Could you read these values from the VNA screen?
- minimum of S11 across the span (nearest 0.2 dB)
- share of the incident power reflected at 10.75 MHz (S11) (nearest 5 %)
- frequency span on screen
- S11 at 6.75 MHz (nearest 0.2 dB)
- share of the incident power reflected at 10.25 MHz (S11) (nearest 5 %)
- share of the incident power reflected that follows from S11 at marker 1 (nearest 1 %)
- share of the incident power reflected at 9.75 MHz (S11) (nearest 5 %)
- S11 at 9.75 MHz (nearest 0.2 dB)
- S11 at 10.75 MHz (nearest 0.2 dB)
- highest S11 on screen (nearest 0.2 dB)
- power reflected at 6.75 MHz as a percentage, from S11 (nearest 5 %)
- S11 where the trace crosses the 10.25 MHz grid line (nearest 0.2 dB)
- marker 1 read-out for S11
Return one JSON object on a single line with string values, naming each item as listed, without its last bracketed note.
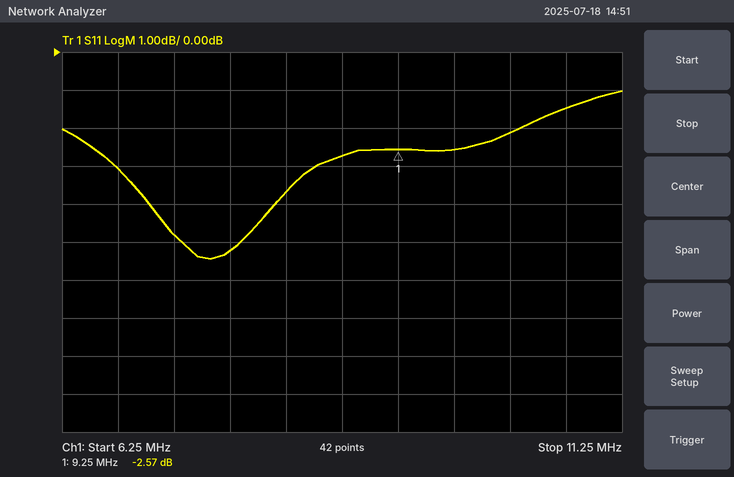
{"minimum of S11 across the span": "-5.4 dB", "share of the incident power reflected at 10.75 MHz (S11)": "70 %", "frequency span on screen": "5 MHz", "S11 at 6.75 MHz": "-3.0 dB", "share of the incident power reflected at 10.25 MHz (S11)": "60 %", "share of the incident power reflected that follows from S11 at marker 1": "55 %", "share of the incident power reflected at 9.75 MHz (S11)": "55 %", "S11 at 9.75 MHz": "-2.6 dB", "S11 at 10.75 MHz": "-1.4 dB", "highest S11 on screen": "-1.0 dB", "power reflected at 6.75 MHz as a percentage, from S11": "50 %", "S11 where the trace crosses the 10.25 MHz grid line": "-2.2 dB", "marker 1 read-out for S11": "-2.57 dB"}
